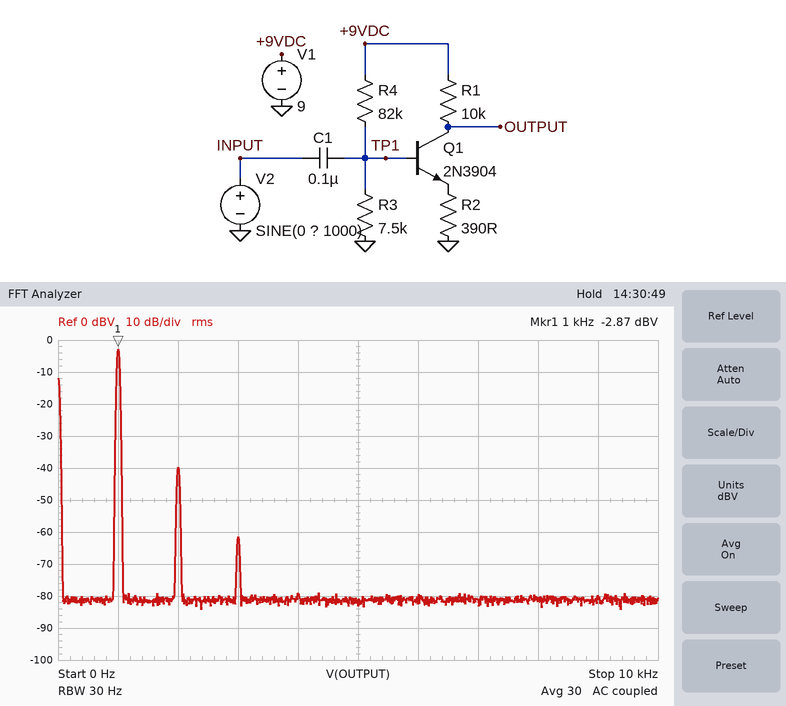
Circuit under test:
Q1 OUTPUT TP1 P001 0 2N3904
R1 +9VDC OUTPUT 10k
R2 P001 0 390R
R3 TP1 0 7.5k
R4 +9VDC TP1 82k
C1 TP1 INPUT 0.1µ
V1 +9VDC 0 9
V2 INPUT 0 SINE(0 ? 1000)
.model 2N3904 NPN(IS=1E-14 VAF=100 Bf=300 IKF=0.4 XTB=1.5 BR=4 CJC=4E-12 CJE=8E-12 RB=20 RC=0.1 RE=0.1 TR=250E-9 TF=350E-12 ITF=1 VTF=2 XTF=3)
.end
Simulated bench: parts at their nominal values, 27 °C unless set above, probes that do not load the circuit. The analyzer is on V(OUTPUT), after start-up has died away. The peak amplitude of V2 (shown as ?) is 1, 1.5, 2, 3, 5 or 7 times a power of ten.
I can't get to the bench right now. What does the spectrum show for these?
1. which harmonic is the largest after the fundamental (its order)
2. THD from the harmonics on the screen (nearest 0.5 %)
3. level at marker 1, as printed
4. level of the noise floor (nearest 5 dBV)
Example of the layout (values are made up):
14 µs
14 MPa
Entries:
2
1.5 %
-2.87 dBV
-80 dBV
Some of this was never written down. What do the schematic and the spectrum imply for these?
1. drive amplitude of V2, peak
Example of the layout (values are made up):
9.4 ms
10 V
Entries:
50 mV
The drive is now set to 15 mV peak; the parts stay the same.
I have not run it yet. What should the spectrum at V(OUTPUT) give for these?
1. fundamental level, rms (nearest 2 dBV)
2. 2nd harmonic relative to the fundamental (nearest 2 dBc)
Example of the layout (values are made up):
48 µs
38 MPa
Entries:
-14 dBV
-48 dBc
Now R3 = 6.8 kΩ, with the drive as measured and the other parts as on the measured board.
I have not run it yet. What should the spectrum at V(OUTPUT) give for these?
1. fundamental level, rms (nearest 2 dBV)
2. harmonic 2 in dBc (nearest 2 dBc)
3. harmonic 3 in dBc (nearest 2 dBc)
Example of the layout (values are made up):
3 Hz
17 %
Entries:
-4 dBV
-30 dBc
-50 dBc
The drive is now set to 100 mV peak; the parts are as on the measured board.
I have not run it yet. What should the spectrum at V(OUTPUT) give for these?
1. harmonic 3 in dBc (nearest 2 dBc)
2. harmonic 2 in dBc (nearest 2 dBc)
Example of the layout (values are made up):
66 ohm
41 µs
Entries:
-46 dBc
-30 dBc
